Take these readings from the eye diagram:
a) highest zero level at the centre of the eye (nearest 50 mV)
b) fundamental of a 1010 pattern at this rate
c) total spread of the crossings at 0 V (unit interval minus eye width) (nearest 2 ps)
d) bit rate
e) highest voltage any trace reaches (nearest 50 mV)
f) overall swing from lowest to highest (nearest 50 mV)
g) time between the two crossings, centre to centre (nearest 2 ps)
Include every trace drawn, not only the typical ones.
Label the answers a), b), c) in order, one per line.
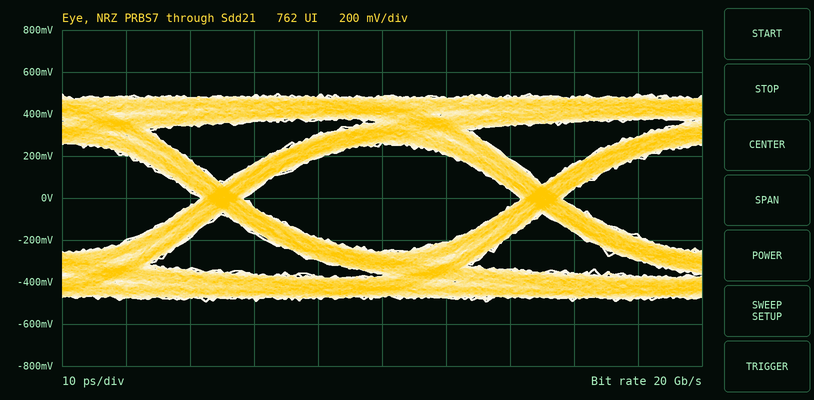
a) -250 mV
b) 10 GHz
c) 6 ps
d) 20 Gb/s
e) 500 mV
f) 1.00 V
g) 50 ps
